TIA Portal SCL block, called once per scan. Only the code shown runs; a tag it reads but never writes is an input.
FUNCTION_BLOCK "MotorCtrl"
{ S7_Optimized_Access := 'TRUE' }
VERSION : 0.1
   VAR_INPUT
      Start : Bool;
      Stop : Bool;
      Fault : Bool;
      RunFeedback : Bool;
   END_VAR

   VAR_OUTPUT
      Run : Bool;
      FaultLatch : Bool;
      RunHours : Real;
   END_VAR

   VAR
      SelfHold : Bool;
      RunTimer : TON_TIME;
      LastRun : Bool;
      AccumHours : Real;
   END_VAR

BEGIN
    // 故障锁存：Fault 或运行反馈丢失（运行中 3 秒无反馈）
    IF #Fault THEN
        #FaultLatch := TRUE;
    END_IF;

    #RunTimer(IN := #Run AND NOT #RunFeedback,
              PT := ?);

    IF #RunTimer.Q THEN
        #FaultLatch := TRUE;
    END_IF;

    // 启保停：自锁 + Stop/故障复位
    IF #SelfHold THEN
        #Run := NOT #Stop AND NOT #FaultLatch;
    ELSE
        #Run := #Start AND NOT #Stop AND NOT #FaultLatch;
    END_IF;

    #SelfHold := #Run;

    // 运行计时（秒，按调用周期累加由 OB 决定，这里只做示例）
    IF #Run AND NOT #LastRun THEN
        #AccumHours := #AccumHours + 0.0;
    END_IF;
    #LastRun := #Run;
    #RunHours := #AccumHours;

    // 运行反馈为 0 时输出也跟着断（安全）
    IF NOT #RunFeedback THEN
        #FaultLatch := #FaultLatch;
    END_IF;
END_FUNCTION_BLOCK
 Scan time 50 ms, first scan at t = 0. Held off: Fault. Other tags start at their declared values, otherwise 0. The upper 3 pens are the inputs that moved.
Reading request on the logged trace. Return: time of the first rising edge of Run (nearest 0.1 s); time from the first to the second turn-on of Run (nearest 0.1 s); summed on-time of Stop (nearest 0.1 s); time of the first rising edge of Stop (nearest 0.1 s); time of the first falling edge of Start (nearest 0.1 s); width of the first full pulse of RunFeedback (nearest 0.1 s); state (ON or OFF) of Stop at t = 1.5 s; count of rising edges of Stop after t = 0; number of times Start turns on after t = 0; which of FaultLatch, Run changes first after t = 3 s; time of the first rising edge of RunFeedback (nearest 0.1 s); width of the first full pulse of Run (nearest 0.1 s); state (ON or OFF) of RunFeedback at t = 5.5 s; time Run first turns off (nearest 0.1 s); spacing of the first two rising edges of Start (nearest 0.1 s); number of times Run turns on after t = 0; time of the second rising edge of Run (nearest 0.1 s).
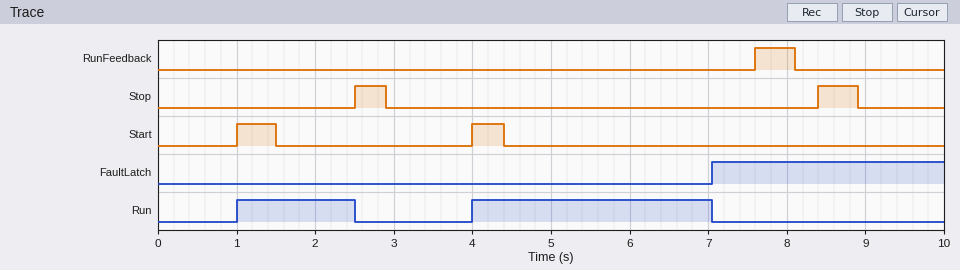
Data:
1.0 s
3.0 s
0.9 s
2.5 s
1.5 s
0.5 s
OFF
2
2
Run
7.6 s
1.5 s
OFF
2.5 s
3.0 s
2
4.0 s
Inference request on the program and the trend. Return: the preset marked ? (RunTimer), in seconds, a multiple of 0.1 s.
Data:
3.0 s
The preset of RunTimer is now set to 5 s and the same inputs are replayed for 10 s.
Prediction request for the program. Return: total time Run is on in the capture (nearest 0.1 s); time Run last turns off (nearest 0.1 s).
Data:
5.9 s
8.4 s
